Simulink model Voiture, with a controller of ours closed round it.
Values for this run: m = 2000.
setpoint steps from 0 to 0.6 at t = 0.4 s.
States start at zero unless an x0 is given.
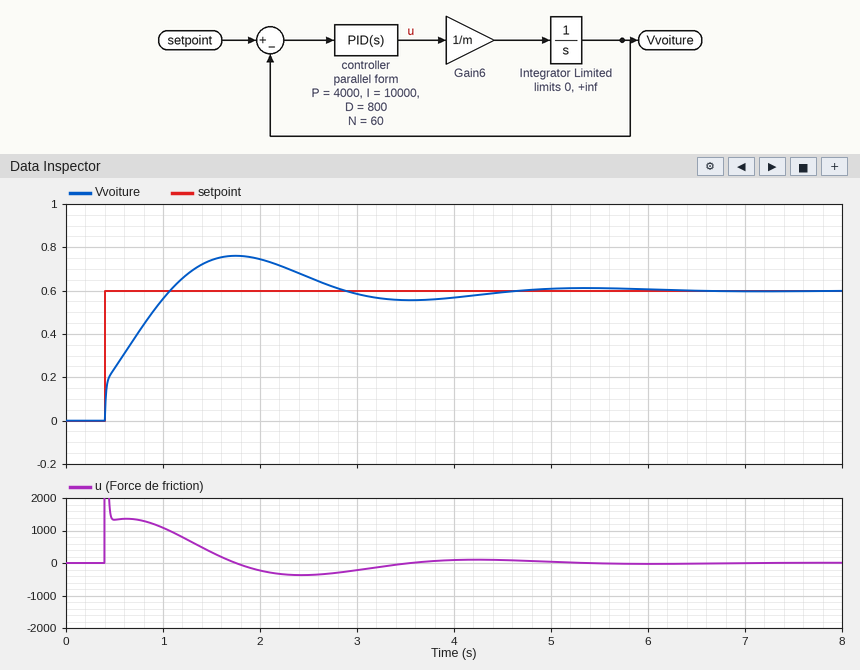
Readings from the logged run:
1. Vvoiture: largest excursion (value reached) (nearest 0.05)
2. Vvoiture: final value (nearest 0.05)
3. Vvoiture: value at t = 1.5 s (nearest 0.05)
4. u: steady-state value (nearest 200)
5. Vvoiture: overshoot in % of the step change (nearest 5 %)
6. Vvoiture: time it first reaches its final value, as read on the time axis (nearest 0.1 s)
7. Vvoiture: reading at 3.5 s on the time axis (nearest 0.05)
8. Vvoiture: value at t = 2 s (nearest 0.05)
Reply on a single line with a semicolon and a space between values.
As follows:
0.75; 0.60; 0.75; 0; 25 %; 1.1 s; 0.55; 0.75
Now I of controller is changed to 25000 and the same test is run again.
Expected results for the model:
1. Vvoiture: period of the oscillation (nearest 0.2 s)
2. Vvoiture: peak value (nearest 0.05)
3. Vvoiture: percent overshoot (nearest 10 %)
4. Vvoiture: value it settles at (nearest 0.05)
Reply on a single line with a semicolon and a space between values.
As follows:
2.2 s; 0.80; 40 %; 0.60
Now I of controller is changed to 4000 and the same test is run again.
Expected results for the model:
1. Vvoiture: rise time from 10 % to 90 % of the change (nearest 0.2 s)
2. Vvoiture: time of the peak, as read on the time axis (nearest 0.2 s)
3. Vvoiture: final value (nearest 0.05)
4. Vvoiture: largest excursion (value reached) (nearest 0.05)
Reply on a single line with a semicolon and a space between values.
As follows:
0.8 s; 2.4 s; 0.60; 0.70
